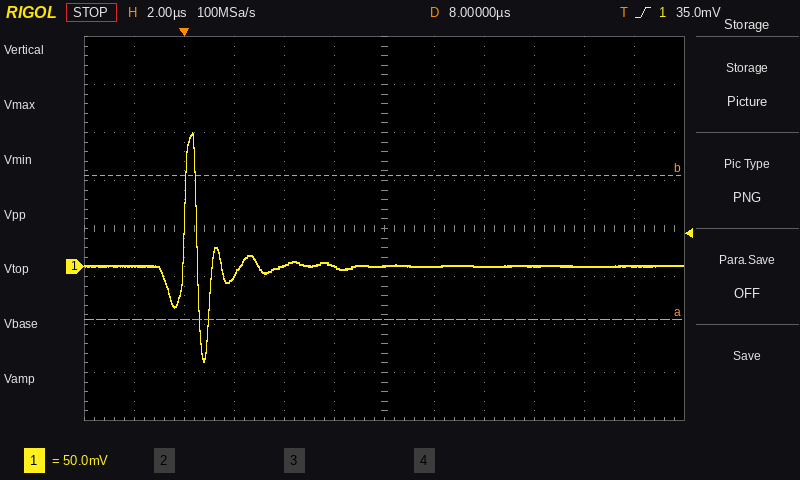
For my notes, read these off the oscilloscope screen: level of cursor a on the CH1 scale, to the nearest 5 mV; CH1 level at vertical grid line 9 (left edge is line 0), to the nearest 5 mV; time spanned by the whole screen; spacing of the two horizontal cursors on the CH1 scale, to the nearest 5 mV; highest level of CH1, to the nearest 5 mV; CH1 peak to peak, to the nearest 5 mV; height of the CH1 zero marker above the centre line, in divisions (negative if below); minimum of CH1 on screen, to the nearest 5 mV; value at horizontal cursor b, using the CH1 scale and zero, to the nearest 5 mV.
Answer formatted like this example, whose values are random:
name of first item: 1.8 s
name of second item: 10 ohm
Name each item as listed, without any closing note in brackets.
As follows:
level of cursor a on the CH1 scale, to the nearest 5 mV: -55 mV
CH1 level at vertical grid line 9 (left edge is line 0), to the nearest 5 mV: 0 mV
time spanned by the whole screen: 24 µs
spacing of the two horizontal cursors on the CH1 scale, to the nearest 5 mV: 150 mV
highest level of CH1, to the nearest 5 mV: 140 mV
CH1 peak to peak, to the nearest 5 mV: 240 mV
height of the CH1 zero marker above the centre line, in divisions: -0.8 div
minimum of CH1 on screen, to the nearest 5 mV: -100 mV
value at horizontal cursor b, using the CH1 scale and zero, to the nearest 5 mV: 95 mV
